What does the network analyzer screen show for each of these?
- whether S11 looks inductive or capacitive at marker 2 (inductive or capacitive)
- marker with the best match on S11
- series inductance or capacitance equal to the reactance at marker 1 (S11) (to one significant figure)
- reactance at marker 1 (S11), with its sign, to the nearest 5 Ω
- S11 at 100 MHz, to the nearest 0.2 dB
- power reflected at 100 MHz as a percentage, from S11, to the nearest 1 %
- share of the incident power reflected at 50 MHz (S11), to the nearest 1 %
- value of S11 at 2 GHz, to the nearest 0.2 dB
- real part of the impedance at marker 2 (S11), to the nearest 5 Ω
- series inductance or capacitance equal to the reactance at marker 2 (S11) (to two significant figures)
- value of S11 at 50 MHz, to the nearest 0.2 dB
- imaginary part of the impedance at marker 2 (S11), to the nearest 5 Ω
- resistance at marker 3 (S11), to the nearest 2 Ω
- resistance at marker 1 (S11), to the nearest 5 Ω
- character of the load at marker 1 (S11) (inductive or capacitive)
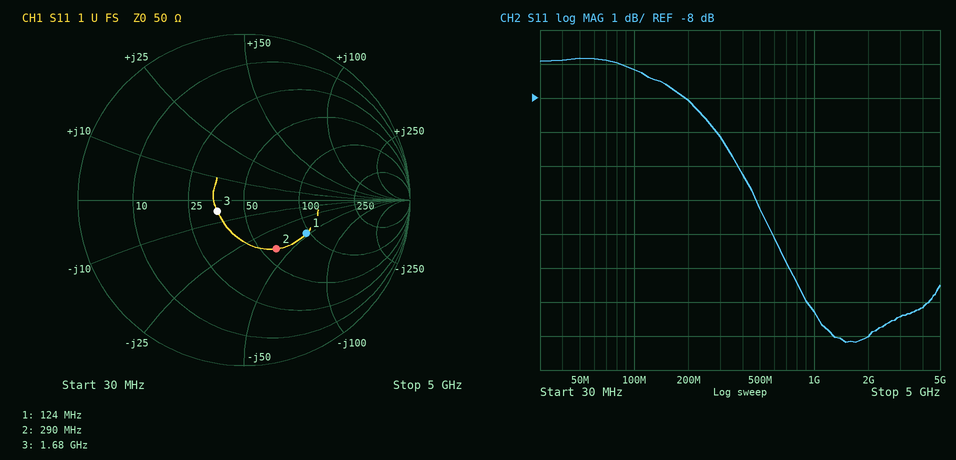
capacitive
marker 3
30 pF
-45 Ω
-7.2 dB
19 %
21 %
-15.0 dB
60 Ω
14 pF
-6.8 dB
-40 Ω
36 Ω
95 Ω
capacitive
